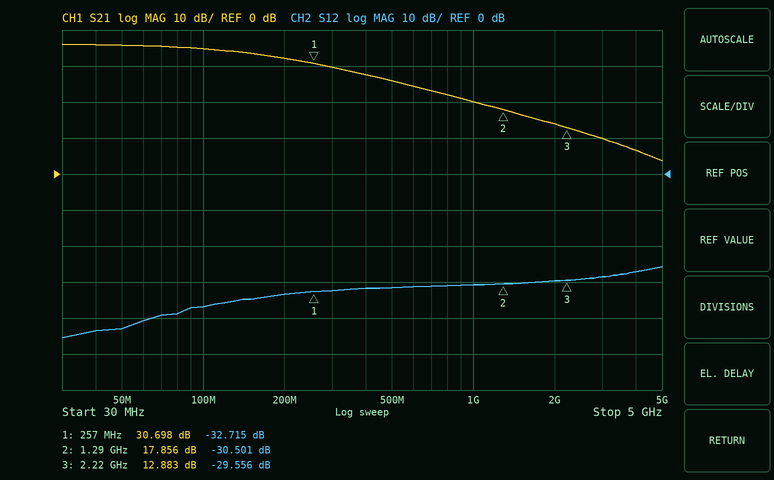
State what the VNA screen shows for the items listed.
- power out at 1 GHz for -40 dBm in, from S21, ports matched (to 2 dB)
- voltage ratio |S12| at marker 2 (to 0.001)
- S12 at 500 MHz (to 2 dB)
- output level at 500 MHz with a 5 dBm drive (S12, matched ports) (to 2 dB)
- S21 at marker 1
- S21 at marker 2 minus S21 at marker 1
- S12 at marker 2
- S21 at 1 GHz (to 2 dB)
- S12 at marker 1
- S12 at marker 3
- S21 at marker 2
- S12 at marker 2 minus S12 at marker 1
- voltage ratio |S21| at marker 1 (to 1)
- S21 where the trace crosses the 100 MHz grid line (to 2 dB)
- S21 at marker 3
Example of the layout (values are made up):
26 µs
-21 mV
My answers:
-20 dBm
0.030
-32 dB
-26 dBm
30.698 dB
-12.842 dB
-30.501 dB
20 dB
-32.715 dB
-29.556 dB
17.856 dB
2.214 dB
34
34 dB
12.883 dB
